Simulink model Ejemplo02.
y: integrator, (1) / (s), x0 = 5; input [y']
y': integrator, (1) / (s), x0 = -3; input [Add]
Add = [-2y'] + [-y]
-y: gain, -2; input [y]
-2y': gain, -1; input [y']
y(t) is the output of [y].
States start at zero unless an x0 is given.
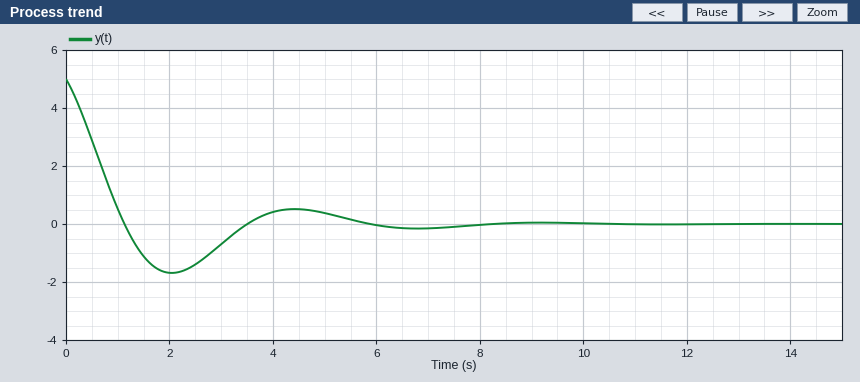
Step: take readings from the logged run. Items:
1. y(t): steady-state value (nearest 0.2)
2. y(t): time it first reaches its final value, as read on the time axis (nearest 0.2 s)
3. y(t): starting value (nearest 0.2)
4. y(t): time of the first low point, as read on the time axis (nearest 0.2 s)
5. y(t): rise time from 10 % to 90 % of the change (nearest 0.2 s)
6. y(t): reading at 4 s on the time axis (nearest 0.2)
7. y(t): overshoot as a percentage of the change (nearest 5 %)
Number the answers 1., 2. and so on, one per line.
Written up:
1. 0.0
2. 1.2 s
3. 5.0
4. 2.0 s
5. 0.8 s
6. 0.4
7. 35 %
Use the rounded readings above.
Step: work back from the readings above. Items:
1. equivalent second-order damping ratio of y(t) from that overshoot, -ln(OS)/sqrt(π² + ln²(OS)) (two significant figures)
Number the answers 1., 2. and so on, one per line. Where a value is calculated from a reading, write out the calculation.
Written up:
1. ln(0.35) = -1.050; 1.050 / sqrt(9.870 + 1.102) = 0.32
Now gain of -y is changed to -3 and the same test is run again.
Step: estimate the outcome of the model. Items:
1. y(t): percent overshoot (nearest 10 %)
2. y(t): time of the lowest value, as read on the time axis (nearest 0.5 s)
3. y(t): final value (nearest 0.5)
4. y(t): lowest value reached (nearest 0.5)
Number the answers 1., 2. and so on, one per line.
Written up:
1. 40 %
2. 1.5 s
3. 0.0
4. -2.0
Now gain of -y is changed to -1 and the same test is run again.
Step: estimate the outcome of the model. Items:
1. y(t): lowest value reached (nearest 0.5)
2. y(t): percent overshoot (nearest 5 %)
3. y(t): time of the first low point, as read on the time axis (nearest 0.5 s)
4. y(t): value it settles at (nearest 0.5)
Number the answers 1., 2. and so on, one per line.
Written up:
1. -1.0
2. 20 %
3. 3.0 s
4. 0.0
